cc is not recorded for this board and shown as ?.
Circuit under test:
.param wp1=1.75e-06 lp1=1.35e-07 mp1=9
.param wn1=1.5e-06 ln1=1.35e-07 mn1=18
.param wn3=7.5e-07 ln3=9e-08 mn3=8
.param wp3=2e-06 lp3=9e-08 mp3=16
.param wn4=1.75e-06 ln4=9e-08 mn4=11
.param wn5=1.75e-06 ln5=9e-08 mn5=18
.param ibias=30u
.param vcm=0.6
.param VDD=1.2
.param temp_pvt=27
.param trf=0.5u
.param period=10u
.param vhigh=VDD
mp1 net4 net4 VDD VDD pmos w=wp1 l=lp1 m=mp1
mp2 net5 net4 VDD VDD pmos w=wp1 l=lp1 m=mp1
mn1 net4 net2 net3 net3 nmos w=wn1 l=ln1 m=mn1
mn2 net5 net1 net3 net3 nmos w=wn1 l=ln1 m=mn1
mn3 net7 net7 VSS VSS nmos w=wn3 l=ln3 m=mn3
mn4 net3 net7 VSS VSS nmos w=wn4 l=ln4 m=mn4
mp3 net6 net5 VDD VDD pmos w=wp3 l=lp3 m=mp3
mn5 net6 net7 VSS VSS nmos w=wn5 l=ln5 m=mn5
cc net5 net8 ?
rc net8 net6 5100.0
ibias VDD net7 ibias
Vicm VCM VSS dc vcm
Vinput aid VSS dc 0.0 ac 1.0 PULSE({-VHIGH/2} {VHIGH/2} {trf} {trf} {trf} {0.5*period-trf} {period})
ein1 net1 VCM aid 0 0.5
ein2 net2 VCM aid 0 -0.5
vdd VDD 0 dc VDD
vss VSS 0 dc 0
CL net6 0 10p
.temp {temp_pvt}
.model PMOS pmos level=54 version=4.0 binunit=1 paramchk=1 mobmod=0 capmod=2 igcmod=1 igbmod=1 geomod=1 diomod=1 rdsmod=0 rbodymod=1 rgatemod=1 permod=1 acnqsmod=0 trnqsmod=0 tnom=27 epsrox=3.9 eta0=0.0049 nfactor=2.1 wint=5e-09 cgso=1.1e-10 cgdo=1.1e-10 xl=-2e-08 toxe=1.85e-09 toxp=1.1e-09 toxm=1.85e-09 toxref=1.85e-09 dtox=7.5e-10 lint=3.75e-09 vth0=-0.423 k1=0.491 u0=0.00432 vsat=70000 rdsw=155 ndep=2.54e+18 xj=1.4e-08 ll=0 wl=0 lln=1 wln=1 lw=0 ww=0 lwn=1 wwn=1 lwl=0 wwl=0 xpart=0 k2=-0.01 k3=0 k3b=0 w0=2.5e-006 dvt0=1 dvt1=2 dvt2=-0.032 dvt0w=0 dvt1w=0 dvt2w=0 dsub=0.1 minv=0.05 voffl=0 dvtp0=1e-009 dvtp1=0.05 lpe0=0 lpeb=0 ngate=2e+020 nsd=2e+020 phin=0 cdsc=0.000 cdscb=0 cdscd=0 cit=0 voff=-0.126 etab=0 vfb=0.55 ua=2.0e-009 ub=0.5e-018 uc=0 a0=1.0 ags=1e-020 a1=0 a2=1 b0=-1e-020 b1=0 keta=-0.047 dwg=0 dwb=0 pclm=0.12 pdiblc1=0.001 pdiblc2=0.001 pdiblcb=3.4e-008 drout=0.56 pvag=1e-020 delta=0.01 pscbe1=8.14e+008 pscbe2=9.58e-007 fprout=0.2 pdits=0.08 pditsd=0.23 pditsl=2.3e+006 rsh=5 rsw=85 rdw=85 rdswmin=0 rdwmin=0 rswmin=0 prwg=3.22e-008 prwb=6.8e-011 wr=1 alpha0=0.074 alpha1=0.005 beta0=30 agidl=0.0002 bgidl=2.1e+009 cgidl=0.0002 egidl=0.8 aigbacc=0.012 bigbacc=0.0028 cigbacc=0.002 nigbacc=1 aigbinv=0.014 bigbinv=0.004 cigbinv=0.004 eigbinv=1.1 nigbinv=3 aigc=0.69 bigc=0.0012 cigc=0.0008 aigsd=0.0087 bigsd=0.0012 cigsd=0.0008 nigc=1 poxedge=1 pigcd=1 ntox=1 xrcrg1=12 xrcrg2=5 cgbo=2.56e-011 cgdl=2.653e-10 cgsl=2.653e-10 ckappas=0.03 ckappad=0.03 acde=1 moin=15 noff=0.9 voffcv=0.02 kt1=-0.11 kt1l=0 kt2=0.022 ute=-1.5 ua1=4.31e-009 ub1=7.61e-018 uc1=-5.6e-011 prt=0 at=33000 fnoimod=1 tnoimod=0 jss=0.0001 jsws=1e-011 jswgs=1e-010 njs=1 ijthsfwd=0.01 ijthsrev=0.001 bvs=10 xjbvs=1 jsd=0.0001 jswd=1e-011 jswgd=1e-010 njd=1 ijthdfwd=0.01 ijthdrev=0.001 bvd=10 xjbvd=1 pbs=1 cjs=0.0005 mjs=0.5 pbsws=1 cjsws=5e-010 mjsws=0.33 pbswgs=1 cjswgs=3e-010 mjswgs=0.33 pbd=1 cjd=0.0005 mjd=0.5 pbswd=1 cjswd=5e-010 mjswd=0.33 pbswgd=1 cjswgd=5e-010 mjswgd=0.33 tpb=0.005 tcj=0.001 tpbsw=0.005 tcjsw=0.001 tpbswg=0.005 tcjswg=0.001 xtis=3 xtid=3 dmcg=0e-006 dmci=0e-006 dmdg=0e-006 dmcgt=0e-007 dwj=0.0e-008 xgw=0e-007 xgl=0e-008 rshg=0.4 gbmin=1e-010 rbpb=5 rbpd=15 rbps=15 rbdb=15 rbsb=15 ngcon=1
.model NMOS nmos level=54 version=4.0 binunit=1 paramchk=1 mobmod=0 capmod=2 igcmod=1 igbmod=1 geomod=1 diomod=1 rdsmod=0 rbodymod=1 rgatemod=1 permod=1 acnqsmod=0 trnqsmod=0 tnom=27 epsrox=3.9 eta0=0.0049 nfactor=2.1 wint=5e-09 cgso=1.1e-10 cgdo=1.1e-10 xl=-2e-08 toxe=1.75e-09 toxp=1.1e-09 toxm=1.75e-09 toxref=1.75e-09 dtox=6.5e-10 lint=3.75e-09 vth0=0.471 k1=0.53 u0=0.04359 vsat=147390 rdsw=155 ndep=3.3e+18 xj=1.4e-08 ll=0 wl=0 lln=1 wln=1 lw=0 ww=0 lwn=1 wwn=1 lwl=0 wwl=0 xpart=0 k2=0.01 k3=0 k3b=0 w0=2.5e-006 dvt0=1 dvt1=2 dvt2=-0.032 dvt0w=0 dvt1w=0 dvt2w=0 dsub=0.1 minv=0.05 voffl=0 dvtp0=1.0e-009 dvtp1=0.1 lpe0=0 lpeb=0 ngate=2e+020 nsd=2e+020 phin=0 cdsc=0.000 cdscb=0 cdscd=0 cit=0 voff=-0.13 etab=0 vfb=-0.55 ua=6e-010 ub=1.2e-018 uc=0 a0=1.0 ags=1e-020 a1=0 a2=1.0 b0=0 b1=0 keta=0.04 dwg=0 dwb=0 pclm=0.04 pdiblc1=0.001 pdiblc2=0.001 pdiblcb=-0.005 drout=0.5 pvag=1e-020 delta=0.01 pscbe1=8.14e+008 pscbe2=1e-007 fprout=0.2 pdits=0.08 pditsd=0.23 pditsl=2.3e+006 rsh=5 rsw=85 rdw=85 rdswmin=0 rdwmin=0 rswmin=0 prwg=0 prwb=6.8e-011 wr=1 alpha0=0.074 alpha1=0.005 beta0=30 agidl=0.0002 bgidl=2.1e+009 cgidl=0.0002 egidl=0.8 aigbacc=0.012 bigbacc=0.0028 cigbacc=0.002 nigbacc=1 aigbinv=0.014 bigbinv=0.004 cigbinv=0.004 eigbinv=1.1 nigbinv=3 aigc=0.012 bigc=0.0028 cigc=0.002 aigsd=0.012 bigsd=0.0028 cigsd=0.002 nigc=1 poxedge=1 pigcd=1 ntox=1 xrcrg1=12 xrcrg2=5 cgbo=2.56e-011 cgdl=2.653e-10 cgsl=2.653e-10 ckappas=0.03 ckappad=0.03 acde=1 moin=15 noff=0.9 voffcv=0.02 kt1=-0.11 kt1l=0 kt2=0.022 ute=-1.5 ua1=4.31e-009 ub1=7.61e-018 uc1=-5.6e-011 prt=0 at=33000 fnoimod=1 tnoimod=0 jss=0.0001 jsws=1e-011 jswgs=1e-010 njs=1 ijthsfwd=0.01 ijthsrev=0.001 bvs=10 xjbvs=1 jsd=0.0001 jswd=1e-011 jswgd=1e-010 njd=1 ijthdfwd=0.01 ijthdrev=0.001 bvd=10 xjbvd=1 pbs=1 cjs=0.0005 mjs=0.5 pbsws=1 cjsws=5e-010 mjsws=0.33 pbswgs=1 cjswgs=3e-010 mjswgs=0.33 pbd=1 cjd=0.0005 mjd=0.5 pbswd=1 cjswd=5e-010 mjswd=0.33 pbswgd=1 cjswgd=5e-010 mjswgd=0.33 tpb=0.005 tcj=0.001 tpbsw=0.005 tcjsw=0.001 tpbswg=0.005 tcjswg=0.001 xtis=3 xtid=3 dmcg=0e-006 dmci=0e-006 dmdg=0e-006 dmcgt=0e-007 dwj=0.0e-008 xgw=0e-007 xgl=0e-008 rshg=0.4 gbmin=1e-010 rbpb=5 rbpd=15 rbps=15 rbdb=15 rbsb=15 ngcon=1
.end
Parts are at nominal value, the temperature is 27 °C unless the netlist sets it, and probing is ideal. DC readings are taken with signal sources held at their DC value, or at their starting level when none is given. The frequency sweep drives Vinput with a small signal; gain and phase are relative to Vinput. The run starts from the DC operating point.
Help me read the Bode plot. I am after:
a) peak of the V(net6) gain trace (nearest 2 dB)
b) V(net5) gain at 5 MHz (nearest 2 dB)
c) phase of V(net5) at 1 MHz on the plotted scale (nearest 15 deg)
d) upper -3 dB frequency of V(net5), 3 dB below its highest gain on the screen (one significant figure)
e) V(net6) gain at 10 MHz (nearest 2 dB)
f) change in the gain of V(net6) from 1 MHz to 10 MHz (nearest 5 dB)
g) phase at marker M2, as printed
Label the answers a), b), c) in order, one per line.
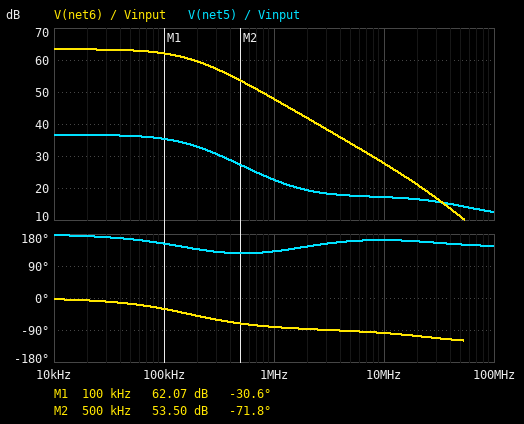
a) 64 dB
b) 18 dB
c) 135 deg
d) 200 kHz
e) 28 dB
f) -20 dB
g) -71.8 deg
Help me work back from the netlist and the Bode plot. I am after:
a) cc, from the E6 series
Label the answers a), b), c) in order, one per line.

a) 470 fF
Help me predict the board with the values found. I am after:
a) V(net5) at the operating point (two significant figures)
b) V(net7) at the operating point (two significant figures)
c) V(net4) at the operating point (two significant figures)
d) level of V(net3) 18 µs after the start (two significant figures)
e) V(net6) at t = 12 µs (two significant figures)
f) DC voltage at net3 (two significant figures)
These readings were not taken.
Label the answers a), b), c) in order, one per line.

a) 680 mV
b) 410 mV
c) 680 mV
d) 470 mV
e) 1.2 V
f) 210 mV
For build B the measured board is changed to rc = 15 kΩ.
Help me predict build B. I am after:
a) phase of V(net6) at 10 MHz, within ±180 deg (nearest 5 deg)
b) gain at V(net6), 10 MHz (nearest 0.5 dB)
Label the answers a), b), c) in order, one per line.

a) -85 deg
b) 28.5 dB
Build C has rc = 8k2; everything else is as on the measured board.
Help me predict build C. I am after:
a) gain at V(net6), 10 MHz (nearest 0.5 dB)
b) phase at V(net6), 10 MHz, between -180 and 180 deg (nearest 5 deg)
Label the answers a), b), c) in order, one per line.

a) 28.0 dB
b) -95 deg
